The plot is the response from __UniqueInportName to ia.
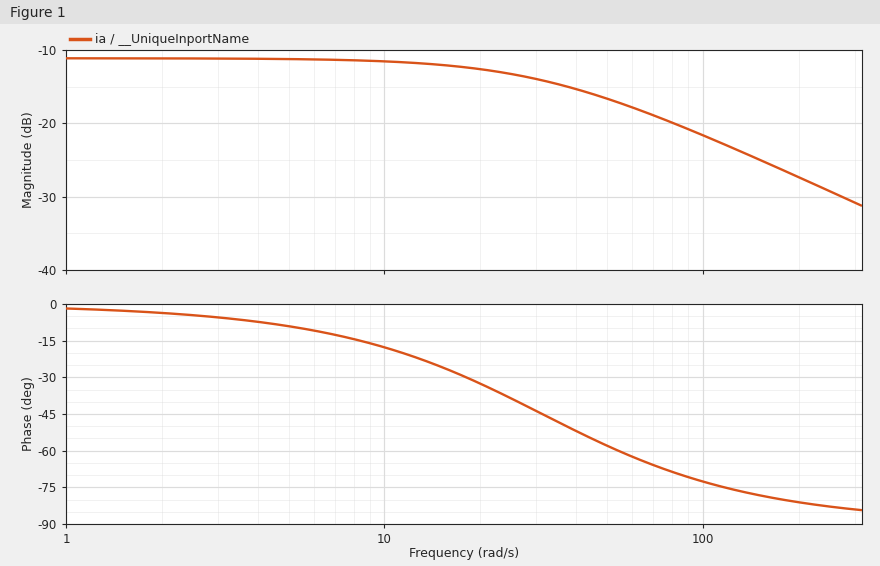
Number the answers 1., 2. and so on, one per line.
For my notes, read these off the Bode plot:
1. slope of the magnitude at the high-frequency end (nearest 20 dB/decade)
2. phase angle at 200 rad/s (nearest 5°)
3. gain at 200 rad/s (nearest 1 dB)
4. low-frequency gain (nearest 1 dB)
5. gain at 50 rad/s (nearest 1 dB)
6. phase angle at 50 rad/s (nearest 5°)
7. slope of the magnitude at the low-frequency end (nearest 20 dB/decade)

1. -20 dB/decade
2. -80°
3. -27 dB
4. -11 dB
5. -17 dB
6. -60°
7. 0 dB/decade
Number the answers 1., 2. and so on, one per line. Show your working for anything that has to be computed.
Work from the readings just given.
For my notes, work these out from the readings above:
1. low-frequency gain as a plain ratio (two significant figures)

1. 10^(-11 / 20) = 0.28
